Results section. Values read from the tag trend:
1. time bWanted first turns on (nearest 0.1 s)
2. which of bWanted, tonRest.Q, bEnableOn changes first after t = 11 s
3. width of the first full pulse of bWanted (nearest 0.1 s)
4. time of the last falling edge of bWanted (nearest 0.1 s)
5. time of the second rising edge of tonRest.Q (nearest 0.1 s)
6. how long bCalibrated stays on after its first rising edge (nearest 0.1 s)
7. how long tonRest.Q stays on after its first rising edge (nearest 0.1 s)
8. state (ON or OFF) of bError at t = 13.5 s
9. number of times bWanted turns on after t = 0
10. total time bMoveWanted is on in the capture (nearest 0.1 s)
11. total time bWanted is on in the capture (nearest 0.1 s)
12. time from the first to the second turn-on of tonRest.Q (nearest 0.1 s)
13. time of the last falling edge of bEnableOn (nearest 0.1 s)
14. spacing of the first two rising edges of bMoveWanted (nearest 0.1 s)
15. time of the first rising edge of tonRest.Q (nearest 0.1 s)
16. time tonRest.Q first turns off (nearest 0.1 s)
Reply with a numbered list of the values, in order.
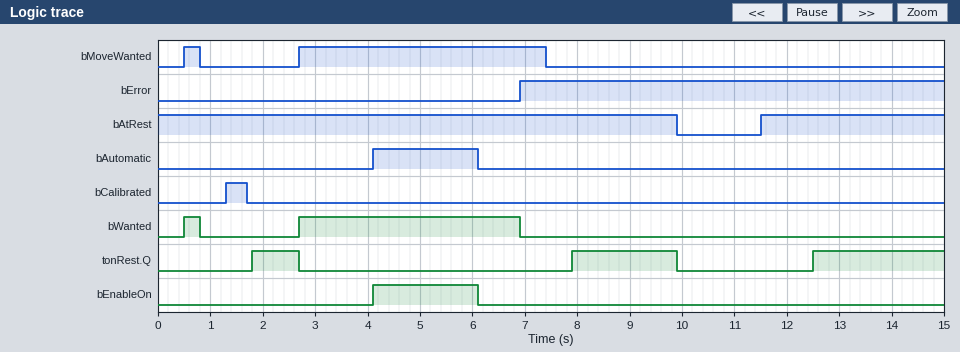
1. 0.5 s
2. tonRest.Q
3. 0.3 s
4. 6.9 s
5. 7.9 s
6. 0.4 s
7. 0.9 s
8. ON
9. 2
10. 5.0 s
11. 4.5 s
12. 6.1 s
13. 6.1 s
14. 2.2 s
15. 1.8 s
16. 2.7 s
